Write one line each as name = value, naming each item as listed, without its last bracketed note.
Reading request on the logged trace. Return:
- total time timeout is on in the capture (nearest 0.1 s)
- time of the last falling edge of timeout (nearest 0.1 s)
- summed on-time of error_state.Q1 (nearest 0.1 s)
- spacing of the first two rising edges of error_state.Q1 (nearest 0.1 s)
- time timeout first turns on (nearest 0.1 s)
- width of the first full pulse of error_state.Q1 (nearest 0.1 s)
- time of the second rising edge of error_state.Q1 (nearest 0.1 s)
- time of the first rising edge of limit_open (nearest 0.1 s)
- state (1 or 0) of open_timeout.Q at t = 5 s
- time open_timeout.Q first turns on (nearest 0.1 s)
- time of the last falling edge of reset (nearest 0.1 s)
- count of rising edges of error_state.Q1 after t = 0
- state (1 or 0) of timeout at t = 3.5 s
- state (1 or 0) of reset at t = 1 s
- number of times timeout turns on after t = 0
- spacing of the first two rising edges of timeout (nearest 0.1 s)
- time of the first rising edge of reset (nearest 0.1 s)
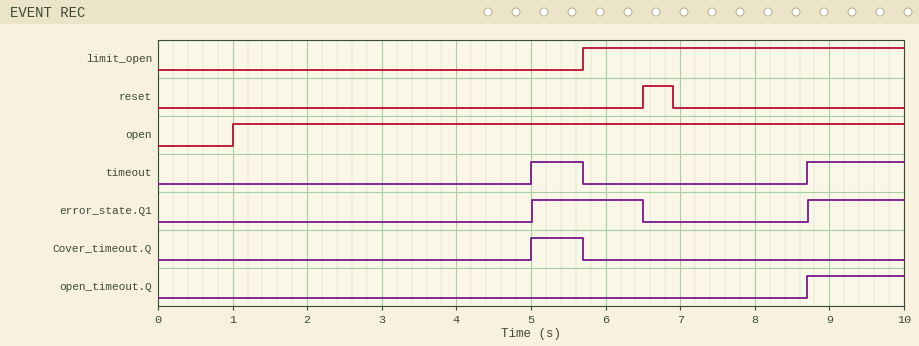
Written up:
total time timeout is on in the capture = 2.0 s
time of the last falling edge of timeout = 5.7 s
summed on-time of error_state.Q1 = 2.8 s
spacing of the first two rising edges of error_state.Q1 = 3.7 s
time timeout first turns on = 5.0 s
width of the first full pulse of error_state.Q1 = 1.5 s
time of the second rising edge of error_state.Q1 = 8.7 s
time of the first rising edge of limit_open = 5.7 s
state (1 or 0) of open_timeout.Q at t = 5 s = 0
time open_timeout.Q first turns on = 8.7 s
time of the last falling edge of reset = 6.9 s
count of rising edges of error_state.Q1 after t = 0 = 2
state (1 or 0) of timeout at t = 3.5 s = 0
state (1 or 0) of reset at t = 1 s = 0
number of times timeout turns on after t = 0 = 2
spacing of the first two rising edges of timeout = 3.7 s
time of the first rising edge of reset = 6.5 s
